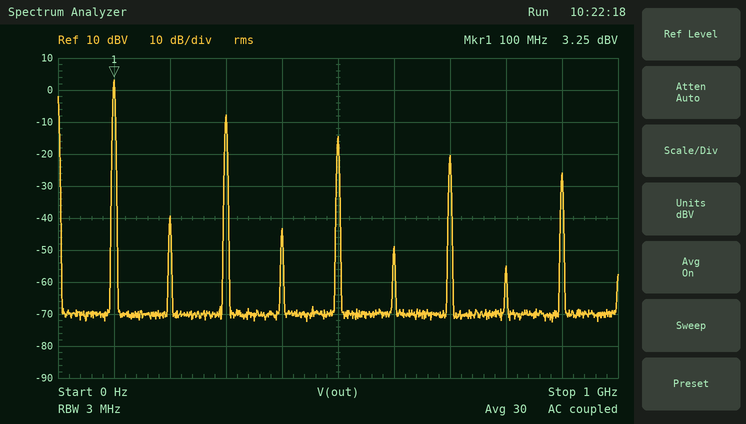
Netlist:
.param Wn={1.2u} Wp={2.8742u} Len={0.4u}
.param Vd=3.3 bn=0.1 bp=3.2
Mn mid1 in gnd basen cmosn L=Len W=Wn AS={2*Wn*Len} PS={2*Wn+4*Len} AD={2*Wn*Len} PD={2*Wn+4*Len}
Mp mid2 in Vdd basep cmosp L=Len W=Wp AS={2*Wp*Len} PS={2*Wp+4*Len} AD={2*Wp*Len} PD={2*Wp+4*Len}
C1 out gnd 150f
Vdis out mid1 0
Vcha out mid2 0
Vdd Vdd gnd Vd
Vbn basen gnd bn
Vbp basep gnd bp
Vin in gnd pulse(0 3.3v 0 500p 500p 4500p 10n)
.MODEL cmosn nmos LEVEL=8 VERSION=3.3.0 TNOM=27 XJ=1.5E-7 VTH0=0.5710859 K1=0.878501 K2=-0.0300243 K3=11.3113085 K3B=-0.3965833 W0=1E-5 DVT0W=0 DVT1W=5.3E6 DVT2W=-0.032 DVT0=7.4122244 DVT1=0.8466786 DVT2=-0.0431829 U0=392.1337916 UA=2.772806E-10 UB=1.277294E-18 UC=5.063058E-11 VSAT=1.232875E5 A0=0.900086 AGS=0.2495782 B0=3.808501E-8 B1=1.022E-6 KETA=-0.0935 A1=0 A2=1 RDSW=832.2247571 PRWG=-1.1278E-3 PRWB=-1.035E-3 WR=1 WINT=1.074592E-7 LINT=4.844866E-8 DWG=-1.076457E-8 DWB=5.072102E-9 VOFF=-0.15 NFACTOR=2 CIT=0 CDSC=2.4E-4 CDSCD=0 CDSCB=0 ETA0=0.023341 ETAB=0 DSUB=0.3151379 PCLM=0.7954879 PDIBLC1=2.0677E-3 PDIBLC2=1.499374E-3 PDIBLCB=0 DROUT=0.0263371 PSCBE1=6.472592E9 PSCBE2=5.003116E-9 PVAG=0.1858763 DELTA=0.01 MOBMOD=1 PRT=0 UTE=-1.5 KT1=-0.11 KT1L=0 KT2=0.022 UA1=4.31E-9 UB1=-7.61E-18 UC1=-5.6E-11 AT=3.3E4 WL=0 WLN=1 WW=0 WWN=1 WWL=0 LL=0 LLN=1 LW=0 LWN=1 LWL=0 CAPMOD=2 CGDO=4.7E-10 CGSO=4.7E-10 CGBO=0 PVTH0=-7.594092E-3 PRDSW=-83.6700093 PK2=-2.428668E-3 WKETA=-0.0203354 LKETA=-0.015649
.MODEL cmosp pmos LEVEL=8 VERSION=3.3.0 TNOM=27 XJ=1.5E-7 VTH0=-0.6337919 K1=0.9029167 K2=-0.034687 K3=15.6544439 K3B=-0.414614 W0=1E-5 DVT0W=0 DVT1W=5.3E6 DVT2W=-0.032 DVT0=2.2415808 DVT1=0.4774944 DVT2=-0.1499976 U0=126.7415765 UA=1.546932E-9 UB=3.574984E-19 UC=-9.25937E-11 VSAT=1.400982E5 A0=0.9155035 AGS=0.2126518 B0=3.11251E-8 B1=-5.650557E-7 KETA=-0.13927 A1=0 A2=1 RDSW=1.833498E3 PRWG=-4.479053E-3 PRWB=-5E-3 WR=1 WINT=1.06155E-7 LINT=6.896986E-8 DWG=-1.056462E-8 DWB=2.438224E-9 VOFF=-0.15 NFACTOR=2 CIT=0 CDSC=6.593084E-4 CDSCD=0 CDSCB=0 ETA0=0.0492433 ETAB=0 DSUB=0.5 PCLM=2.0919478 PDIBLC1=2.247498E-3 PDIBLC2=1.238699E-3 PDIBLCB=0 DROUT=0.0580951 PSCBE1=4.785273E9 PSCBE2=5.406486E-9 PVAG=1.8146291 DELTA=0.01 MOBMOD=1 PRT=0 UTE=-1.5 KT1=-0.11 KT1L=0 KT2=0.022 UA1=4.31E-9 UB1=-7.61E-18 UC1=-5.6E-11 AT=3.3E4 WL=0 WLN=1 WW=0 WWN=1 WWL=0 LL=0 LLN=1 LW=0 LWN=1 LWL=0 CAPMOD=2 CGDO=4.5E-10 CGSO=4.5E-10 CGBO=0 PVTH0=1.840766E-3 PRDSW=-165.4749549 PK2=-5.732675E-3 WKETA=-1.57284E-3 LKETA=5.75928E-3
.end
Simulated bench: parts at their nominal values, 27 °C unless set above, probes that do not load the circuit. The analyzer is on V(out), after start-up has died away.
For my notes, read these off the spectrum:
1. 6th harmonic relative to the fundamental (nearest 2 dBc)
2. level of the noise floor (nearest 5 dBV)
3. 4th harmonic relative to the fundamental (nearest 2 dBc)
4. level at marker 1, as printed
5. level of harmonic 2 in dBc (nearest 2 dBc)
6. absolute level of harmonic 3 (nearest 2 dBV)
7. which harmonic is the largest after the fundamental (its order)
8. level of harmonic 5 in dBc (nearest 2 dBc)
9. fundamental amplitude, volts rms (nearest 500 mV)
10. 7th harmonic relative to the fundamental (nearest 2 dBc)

-52 dBc
-70 dBV
-46 dBc
3.25 dBV
-42 dBc
-8 dBV
3
-18 dBc
1.5 V
-24 dBc
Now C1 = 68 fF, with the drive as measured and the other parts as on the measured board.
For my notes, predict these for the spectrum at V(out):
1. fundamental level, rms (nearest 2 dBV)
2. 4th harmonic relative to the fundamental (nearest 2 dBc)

4 dBV
-44 dBc
